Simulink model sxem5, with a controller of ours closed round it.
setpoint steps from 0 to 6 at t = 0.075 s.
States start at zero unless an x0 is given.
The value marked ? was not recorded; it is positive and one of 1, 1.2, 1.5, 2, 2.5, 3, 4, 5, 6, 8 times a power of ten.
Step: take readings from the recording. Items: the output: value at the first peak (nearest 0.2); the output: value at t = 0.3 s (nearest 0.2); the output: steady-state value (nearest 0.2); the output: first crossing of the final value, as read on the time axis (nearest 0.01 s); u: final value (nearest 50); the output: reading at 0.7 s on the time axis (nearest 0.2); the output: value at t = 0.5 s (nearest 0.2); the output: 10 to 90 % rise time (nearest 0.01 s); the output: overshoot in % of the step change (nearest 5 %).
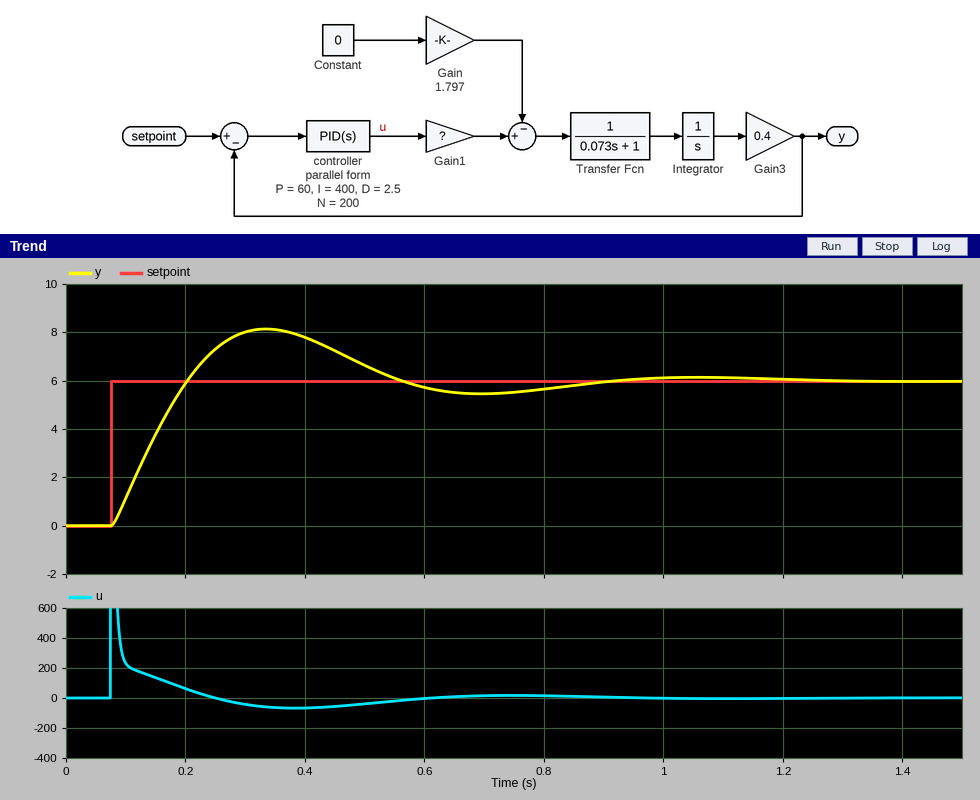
8.2
8.0
6.0
0.20 s
0
5.4
6.6
0.10 s
35 %
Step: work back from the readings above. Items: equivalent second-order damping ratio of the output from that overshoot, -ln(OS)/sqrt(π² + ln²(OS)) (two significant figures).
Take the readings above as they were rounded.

0.32
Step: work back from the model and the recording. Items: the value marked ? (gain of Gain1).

0.6
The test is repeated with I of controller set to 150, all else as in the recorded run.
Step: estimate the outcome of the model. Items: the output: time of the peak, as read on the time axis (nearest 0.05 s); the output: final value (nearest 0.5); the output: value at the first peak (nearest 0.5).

0.35 s
6.0
7.0
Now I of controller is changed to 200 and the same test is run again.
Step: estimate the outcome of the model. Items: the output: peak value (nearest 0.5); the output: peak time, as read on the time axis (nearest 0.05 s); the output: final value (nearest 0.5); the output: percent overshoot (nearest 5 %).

7.5
0.35 s
6.0
20 %
